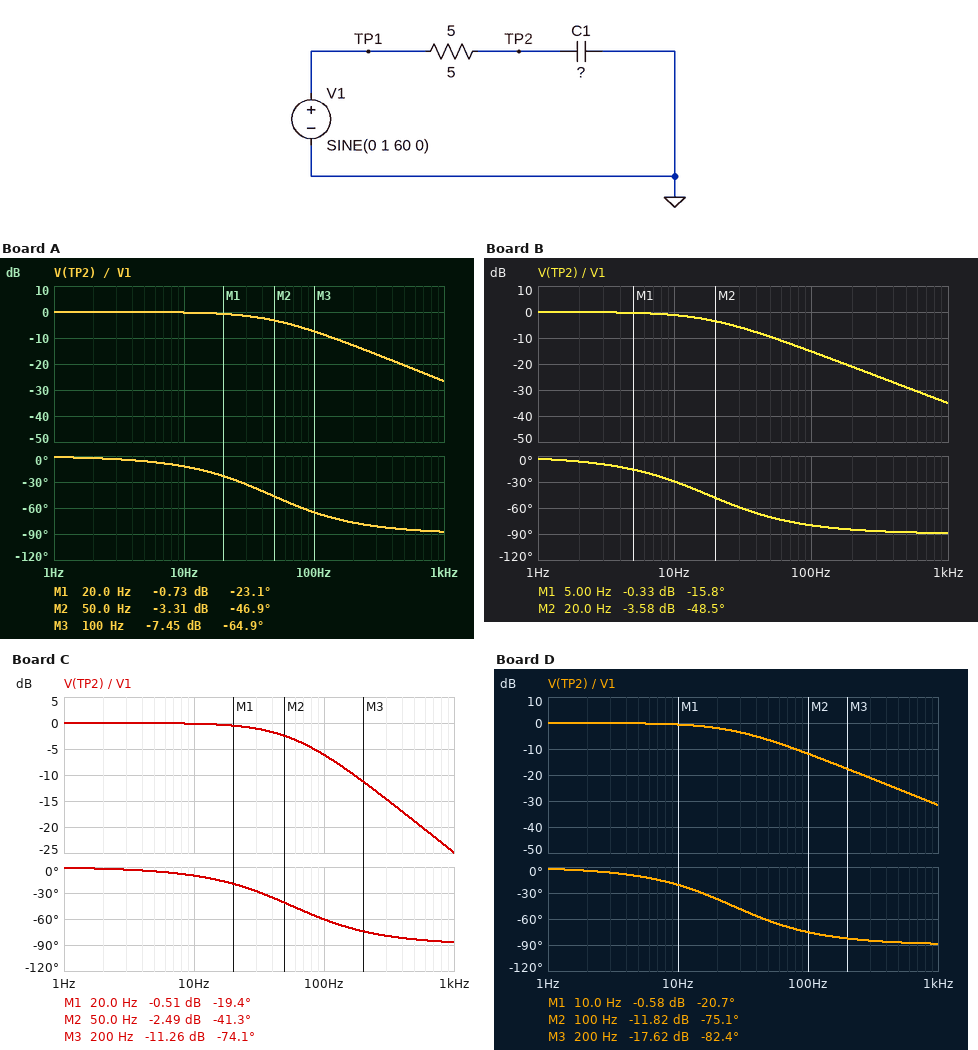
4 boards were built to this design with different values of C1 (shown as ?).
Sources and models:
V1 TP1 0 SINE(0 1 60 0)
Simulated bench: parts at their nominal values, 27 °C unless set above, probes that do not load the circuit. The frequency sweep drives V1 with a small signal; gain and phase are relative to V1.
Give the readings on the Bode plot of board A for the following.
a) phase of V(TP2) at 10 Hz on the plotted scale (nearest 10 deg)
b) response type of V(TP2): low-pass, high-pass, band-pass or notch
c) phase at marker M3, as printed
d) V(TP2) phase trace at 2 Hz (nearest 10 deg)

-10 deg
low-pass
-64.9 deg
0 deg
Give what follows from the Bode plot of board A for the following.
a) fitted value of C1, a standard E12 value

680 µF
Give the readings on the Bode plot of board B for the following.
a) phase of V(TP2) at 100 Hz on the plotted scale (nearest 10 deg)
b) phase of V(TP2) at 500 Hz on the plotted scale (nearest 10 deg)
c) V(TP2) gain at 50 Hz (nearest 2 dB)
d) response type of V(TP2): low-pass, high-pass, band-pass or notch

-80 deg
-90 deg
-10 dB
low-pass
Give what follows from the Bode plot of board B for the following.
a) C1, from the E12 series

1.8 mF
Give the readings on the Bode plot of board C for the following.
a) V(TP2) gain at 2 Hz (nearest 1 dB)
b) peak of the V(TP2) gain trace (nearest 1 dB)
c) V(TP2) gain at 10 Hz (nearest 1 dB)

0 dB
0 dB
0 dB
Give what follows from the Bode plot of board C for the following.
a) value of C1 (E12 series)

560 µF
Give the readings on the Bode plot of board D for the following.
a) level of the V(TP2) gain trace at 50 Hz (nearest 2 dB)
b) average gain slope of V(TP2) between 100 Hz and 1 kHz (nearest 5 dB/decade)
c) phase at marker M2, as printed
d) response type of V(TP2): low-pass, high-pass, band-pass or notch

-6 dB
-20 dB/decade
-75.1 deg
low-pass
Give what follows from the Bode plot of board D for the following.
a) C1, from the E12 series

1.2 mF
